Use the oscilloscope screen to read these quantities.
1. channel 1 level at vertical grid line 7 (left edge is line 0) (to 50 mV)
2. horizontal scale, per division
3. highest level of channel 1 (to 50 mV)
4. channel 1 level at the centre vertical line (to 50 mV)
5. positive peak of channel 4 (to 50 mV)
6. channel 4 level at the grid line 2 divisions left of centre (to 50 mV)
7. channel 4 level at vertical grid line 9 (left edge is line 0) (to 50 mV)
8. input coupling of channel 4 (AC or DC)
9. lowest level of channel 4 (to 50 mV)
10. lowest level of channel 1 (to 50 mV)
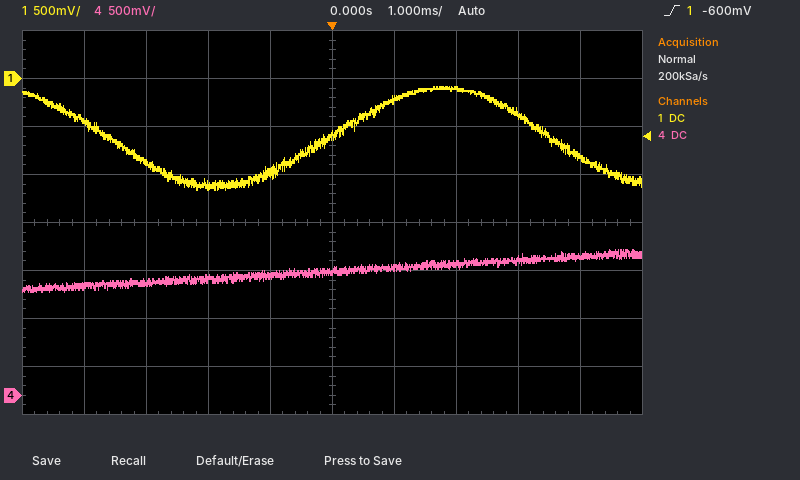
-100 mV
1 ms
-100 mV
-600 mV
1.50 V
1.20 V
1.45 V
DC
1.10 V
-1.15 V
